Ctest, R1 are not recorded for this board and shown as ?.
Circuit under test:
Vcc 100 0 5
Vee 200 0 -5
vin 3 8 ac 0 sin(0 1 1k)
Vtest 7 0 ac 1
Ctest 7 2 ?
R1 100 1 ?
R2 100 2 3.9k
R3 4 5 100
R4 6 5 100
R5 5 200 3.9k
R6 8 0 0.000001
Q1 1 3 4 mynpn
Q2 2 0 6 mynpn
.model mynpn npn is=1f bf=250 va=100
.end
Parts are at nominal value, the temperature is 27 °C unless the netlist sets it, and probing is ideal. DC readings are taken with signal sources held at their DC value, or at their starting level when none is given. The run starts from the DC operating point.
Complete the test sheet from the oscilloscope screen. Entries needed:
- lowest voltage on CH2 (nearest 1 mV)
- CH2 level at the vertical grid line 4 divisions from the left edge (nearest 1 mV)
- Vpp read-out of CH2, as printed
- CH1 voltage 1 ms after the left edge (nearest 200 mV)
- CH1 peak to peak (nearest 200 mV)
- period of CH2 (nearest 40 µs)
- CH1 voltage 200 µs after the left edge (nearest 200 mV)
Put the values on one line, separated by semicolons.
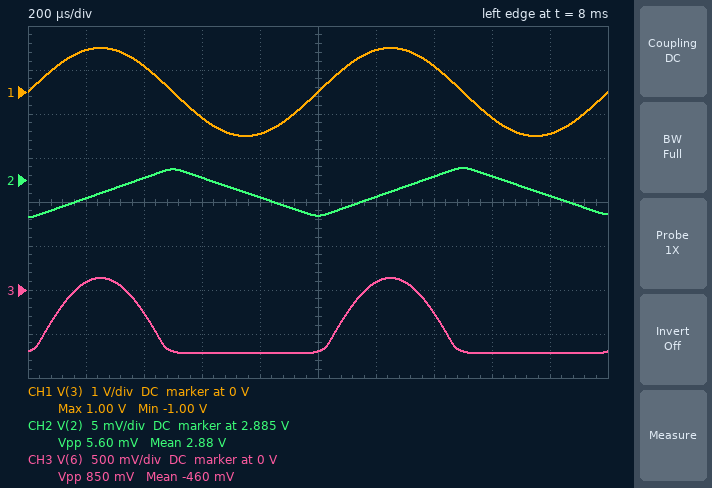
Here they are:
2.881 V; 2.883 V; 5.60 mV; 0 V; 2.0 V; 1.00 ms; 1.0 V
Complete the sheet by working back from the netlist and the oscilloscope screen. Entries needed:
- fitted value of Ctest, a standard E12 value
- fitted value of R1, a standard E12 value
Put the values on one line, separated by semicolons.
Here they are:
47 µF; 6.8 kΩ
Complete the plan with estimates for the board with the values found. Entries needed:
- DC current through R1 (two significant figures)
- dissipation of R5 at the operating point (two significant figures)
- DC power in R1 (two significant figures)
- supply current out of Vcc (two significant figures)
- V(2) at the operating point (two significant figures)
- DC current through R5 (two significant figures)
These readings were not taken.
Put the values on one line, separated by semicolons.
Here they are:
540 µA; 4.6 mW; 2.0 mW; 1.1 mA; 2.9 V; 1.1 mA
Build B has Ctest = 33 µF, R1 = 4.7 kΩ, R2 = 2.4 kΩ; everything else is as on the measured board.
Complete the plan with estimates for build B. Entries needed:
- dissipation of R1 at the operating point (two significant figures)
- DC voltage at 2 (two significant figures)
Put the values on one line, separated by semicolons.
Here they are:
1.4 mW; 3.7 V
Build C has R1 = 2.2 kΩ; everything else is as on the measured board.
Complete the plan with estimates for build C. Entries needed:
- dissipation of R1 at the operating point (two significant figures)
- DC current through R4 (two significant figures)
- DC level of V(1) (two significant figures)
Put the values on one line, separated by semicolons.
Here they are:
650 µW; 540 µA; 3.8 V
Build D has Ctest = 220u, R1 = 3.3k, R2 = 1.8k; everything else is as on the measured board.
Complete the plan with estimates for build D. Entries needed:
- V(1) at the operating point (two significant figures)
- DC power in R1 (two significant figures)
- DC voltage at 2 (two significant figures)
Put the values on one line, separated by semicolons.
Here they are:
3.2 V; 970 µW; 4.0 V
